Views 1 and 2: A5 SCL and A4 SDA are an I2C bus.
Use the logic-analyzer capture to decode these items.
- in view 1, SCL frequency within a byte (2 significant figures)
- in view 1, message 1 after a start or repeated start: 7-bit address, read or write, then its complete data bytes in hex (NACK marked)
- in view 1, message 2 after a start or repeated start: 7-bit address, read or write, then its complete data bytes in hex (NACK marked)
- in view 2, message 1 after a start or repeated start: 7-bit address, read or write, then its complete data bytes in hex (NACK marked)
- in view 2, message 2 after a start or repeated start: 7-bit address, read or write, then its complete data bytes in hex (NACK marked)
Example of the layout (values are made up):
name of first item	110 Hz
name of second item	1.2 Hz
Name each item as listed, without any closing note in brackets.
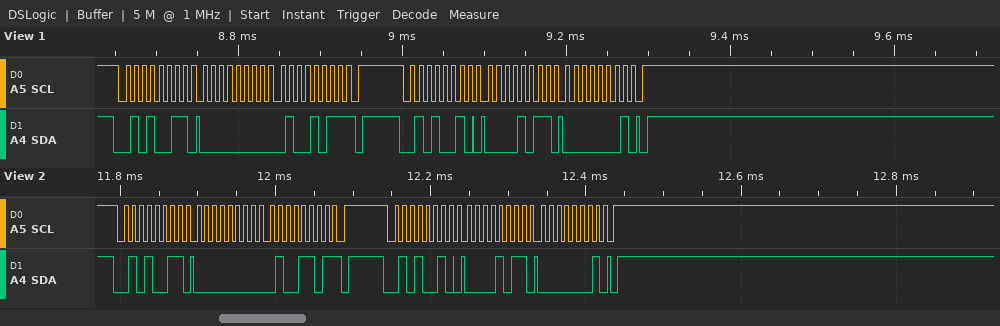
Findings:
in view 1, SCL frequency within a byte	100 kHz
in view 1, message 1 after a start or repeated start: 7-bit address, read or write, then its complete data bytes in hex	0x29 read: 00 4B NACK
in view 1, message 2 after a start or repeated start: 7-bit address, read or write, then its complete data bytes in hex	0x29 write: 0B 01
in view 2, message 1 after a start or repeated start: 7-bit address, read or write, then its complete data bytes in hex	0x29 read: 00 4D NACK
in view 2, message 2 after a start or repeated start: 7-bit address, read or write, then its complete data bytes in hex	0x29 write: 0B 01
